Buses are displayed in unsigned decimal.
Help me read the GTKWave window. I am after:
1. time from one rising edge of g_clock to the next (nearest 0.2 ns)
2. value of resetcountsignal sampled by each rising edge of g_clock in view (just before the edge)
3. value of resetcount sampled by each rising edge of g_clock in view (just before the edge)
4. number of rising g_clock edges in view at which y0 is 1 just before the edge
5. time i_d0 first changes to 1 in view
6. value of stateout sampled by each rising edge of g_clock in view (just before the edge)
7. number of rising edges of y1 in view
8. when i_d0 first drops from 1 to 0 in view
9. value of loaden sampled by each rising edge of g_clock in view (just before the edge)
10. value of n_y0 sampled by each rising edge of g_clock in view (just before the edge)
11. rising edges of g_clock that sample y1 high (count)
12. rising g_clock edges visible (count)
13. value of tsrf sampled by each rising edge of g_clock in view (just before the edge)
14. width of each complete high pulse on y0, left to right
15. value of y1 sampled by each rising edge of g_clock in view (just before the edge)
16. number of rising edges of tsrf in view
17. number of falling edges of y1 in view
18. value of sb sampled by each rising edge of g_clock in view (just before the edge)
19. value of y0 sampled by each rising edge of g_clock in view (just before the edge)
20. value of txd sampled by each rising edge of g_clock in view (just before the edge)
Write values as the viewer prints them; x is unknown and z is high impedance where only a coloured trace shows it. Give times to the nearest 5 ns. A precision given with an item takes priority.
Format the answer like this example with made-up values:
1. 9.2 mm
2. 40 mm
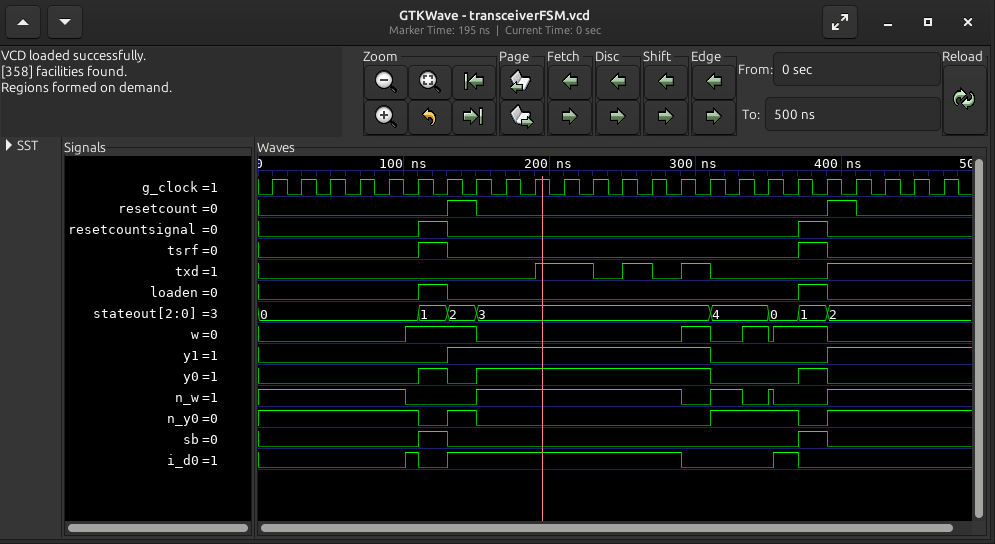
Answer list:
1. 20 ns
2. 0 0 0 0 0 0 1 0 0 0 0 0 0 0 0 0 0 0 0 1 0 0 0 0
3. 0 0 0 0 0 0 0 1 0 0 0 0 0 0 0 0 0 0 0 0 1 0 0 0
4. 10
5. 100 ns
6. 0, 0, 0, 0, 0, 0, 1, 2, 3, 3, 3, 3, 3, 3, 3, 3, 4, 4, 0, 1, 2, 2, 2, 2
7. 2
8. 110 ns
9. 0 0 0 0 0 0 1 0 0 0 0 0 0 0 0 0 0 0 0 1 0 0 0 0
10. 1 1 1 1 1 1 0 1 0 0 0 0 0 0 0 0 1 1 1 0 1 1 1 1
11. 13
12. 24
13. 0 0 0 0 0 0 1 0 0 0 0 0 0 0 0 0 0 0 0 1 0 0 0 0
14. 20 ns, 160 ns, 20 ns
15. 0 0 0 0 0 0 0 1 1 1 1 1 1 1 1 1 0 0 0 0 1 1 1 1
16. 2
17. 1
18. 0 0 0 0 0 0 1 0 0 0 0 0 0 0 0 0 0 0 0 1 0 0 0 0
19. 0 0 0 0 0 0 1 0 1 1 1 1 1 1 1 1 0 0 0 1 0 0 0 0
20. 0 0 0 0 0 0 0 0 0 0 1 1 0 1 0 1 0 0 0 0 1 1 1 1
